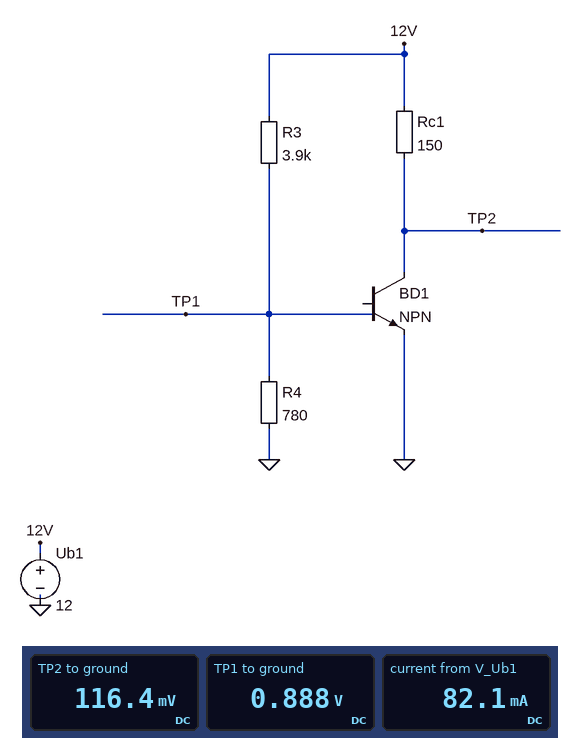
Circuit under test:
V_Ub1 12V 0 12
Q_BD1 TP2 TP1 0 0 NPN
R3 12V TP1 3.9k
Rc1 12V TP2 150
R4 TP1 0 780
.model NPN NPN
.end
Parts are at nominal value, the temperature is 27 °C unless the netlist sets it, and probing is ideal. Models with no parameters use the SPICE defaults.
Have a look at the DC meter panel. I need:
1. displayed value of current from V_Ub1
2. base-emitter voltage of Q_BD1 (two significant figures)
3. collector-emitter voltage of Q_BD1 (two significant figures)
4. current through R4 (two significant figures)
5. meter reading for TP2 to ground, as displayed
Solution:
82.1 mA
890 mV
120 mV
1.1 mA
116.4 mV
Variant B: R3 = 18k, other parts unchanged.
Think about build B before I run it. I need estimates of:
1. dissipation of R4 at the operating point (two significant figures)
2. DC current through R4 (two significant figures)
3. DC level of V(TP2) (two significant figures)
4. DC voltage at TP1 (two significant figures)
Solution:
320 µW
640 µA
12 V
500 mV
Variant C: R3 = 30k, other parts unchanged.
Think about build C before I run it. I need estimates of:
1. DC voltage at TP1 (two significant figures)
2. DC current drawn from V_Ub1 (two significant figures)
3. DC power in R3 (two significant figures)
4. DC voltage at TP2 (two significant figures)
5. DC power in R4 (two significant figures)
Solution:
300 mV
390 µA
4.6 mW
12 V
120 µW
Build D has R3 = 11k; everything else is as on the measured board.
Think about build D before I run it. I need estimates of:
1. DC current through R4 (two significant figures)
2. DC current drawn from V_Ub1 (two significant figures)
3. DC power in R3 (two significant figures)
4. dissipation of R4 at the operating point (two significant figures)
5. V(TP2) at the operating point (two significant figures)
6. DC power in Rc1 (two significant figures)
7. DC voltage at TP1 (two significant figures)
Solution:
1.0 mA
2.5 mA
11 mW
790 µW
12 V
320 µW
780 mV
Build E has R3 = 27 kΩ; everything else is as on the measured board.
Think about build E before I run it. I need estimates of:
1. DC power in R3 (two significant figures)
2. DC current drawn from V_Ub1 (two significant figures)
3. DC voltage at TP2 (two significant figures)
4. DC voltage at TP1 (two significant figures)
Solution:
5.0 mW
430 µA
12 V
340 mV
